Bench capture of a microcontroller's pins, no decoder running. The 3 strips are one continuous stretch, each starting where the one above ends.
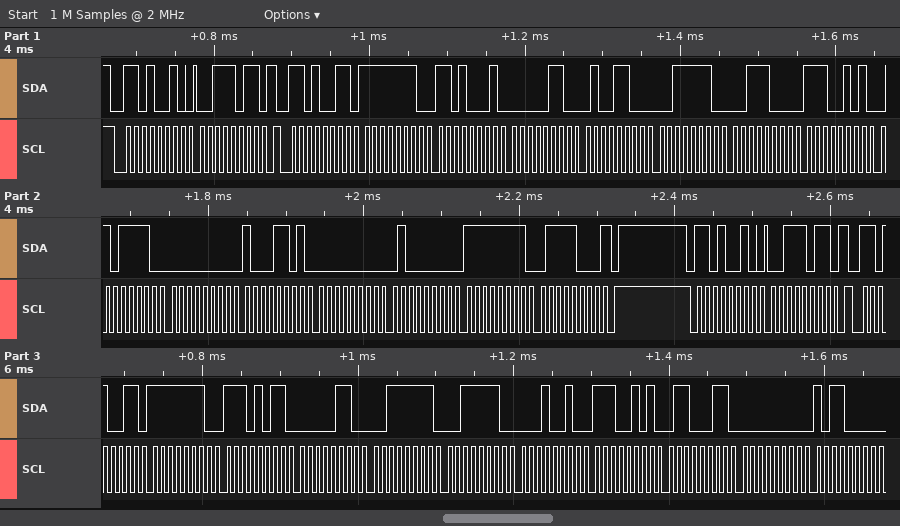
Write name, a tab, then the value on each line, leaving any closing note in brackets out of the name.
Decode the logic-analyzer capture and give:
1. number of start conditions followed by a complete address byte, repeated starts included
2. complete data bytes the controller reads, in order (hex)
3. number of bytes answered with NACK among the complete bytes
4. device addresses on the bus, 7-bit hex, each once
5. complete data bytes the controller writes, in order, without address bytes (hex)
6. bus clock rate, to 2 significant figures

number of start conditions followed by a complete address byte, repeated starts included	4
complete data bytes the controller reads, in order	FE D1 06 4C 3E 38 E5 5E 00 8D 00 40 FF 78 FE EB 06 3F 3E 12 E5 63 00 B0
number of bytes answered with NACK among the complete bytes	1
device addresses on the bus, 7-bit hex, each once	0x69
complete data bytes the controller writes, in order, without address bytes	3B 3B
bus clock rate, to 2 significant figures	100 kHz
